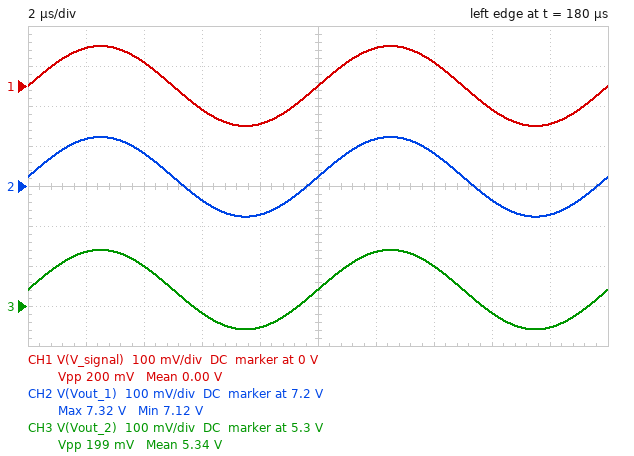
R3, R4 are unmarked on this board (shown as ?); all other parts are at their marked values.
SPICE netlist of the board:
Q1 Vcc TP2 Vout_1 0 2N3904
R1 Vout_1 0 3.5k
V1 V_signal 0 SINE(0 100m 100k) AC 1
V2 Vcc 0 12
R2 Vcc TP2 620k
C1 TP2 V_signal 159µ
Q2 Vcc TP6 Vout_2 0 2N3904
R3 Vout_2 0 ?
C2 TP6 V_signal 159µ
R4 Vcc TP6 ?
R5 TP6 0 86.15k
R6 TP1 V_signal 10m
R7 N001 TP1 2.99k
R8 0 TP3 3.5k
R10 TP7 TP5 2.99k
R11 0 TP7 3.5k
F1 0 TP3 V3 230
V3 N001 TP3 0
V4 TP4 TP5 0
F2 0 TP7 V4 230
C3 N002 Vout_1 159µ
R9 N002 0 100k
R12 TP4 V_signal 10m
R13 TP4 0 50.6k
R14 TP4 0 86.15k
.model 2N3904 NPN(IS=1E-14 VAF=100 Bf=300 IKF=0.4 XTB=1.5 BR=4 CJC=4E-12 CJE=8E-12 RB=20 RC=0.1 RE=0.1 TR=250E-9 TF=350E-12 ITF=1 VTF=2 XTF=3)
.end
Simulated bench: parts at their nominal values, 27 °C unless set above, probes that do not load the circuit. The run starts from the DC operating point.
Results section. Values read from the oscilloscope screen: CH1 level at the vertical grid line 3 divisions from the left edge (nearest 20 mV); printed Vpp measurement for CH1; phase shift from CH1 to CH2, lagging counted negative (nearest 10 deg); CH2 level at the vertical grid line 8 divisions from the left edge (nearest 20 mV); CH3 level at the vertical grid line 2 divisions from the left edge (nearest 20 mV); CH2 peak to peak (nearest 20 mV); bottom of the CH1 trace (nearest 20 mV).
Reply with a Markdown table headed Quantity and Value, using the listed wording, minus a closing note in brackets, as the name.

| Quantity | Value |
|---|---|
| CH1 level at the vertical grid line 3 divisions from the left edge | -60 mV |
| printed Vpp measurement for CH1 | 200 mV |
| phase shift from CH1 to CH2, lagging counted negative | 0 deg |
| CH2 level at the vertical grid line 8 divisions from the left edge | 7.16 V |
| CH3 level at the vertical grid line 2 divisions from the left edge | 5.40 V |
| CH2 peak to peak | 200 mV |
| bottom of the CH1 trace | -100 mV |
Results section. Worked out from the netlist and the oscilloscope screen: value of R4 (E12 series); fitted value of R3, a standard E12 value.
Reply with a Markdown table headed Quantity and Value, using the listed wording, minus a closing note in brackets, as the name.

| Quantity | Value |
|---|---|
| value of R4 | 82 kΩ |
| fitted value of R3, a standard E12 value | 4.7 kΩ |
